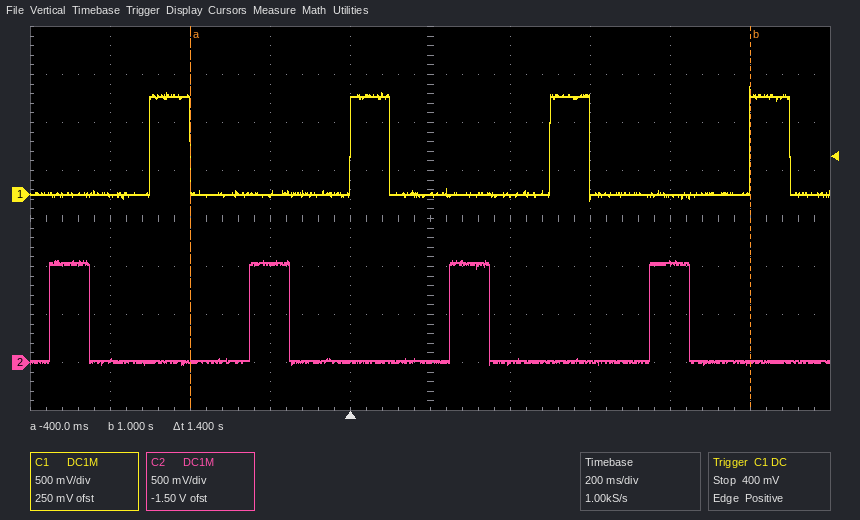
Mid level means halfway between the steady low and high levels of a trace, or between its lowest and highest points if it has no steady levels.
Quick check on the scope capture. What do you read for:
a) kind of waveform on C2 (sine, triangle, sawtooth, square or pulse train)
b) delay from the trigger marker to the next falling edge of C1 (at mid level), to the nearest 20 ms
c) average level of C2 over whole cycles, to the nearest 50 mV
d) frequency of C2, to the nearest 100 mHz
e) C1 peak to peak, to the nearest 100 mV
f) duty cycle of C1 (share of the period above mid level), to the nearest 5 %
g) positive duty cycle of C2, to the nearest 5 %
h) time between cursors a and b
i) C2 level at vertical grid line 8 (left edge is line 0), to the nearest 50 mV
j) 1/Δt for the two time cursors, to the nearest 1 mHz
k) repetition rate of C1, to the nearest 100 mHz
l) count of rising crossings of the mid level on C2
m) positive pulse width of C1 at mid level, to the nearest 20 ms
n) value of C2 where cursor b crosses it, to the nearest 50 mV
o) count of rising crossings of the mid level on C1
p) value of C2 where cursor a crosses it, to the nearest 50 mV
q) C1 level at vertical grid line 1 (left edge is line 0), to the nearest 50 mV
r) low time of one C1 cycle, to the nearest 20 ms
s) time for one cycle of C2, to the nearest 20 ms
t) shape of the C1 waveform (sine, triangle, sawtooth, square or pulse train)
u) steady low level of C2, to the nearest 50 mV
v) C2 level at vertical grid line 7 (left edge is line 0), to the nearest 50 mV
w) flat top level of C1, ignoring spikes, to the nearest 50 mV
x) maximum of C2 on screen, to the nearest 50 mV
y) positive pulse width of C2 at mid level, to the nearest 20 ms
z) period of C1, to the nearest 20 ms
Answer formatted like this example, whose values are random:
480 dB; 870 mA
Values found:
pulse train; 100 ms; 200 mV; 2.0 Hz; 1.20 V; 20 %; 20 %; 1.4 s; 1.05 V; 714 mHz; 2.0 Hz; 4; 100 ms; 0 mV; 4; 0 mV; 0 mV; 400 ms; 500 ms; pulse train; 0 mV; 0 mV; 1.00 V; 1.05 V; 100 ms; 500 ms
